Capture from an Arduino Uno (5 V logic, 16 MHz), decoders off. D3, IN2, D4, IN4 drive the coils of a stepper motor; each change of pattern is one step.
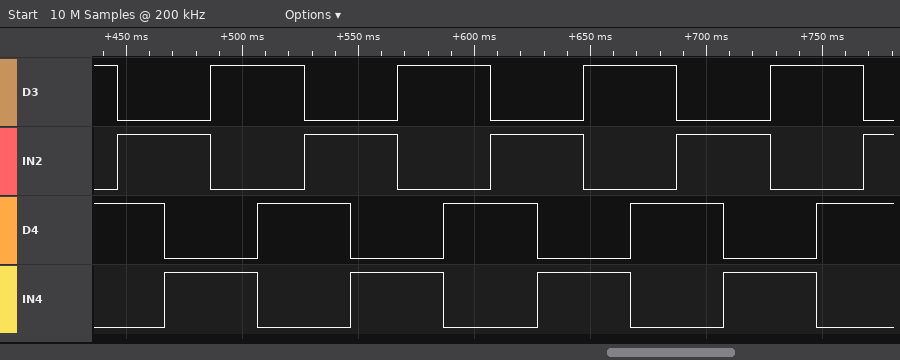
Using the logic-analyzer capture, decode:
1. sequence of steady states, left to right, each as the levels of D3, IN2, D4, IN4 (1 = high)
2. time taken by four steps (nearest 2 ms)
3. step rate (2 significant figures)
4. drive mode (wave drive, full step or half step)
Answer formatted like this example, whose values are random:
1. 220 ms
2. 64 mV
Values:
1. 1010 0110 0101 1001 1010 0110 0101 1001 1010 0110 0101 1001 1010 0110 0101 1001 1010 0110
2. 80 ms
3. 50 steps/s
4. full step
